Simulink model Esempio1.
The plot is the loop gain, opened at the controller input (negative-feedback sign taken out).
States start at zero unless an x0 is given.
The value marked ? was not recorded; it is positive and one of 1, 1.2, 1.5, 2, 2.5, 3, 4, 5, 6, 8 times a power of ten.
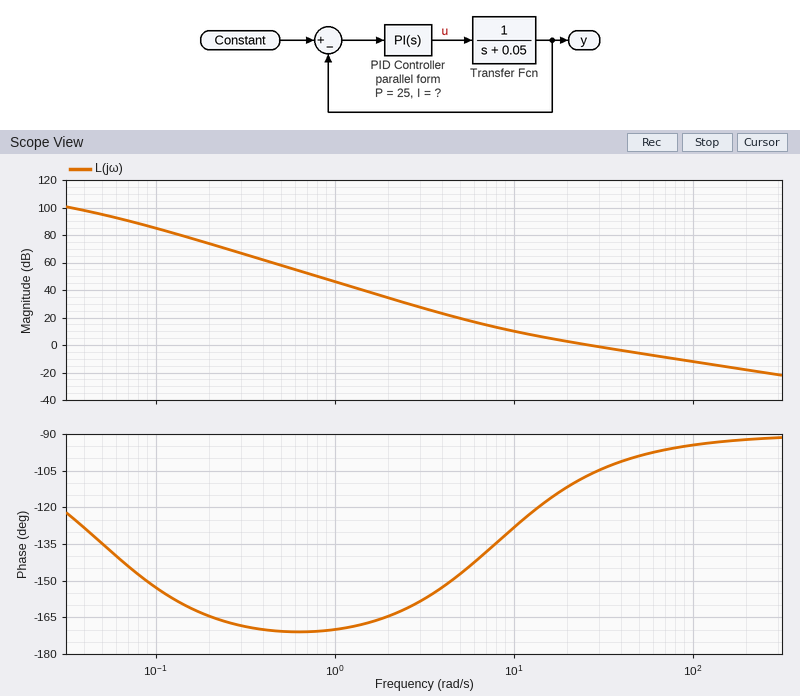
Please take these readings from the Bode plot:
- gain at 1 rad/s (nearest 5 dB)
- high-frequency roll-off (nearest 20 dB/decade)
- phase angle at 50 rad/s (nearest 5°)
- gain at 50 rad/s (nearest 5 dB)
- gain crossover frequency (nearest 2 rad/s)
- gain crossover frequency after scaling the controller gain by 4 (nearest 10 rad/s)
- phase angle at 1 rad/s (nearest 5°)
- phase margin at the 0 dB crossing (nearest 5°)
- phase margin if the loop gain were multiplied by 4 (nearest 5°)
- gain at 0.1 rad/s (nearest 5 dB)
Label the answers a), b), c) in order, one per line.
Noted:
a) 45 dB
b) -20 dB/decade
c) -100°
d) -5 dB
e) 26 rad/s
f) 100 rad/s
g) -170°
h) 75°
i) 85°
j) 85 dB
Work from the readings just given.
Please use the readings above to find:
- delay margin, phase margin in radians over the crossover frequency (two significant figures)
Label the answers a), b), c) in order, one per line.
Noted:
a) 0.050 s
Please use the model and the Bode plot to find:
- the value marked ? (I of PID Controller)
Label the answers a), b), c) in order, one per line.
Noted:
a) 200
